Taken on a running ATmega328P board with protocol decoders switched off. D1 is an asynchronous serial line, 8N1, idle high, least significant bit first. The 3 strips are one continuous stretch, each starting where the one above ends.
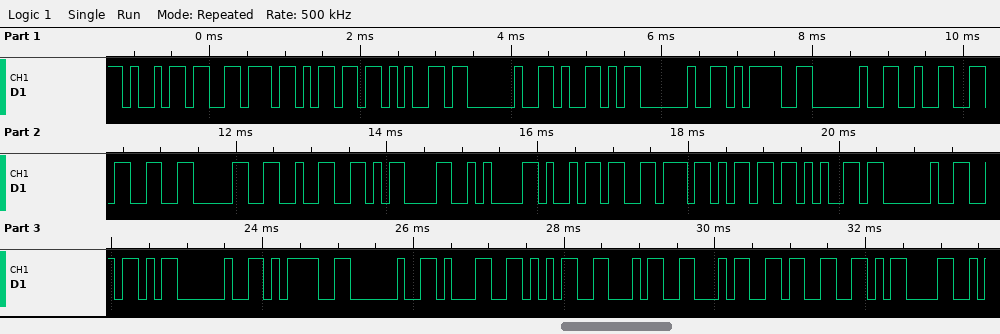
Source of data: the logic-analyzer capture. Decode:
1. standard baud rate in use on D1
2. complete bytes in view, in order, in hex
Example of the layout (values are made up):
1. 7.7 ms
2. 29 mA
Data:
1. 9600 baud
2. 69 76 6D 65 20 59 20 3D 20 32 33 30 32 0D 0A 69 76 6D 65 20 5A 20 3D 20 31 35 34 34 33 0D
